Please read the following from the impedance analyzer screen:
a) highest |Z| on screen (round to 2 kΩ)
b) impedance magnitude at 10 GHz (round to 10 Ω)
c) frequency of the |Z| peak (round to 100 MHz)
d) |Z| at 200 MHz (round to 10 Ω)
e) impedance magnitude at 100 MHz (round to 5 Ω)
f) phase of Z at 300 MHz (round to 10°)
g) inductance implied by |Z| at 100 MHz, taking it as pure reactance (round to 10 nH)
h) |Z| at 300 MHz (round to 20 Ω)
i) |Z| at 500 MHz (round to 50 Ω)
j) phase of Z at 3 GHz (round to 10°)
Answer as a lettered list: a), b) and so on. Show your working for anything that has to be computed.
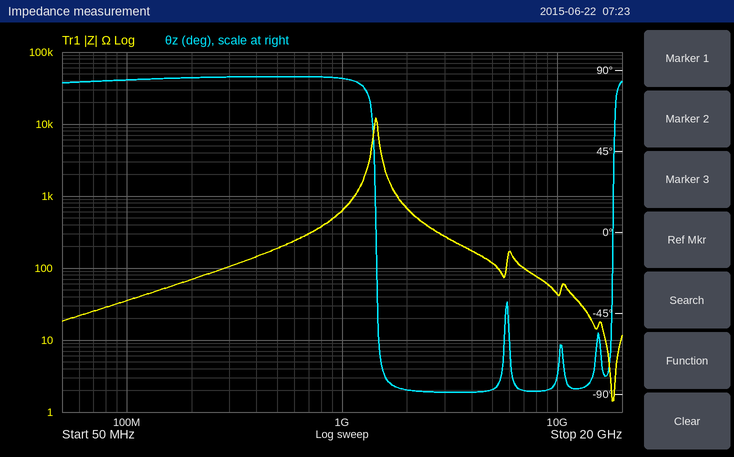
a) 12 kΩ
b) 40 Ω
c) 1.4 GHz
d) 70 Ω
e) 35 Ω
f) 90°
g) L = 35 Ω/(2π × 100 MHz) ≈ 55.7 nH, so 60 nH to the nearest 10 nH
h) 100 Ω
i) 200 Ω
j) -90°
